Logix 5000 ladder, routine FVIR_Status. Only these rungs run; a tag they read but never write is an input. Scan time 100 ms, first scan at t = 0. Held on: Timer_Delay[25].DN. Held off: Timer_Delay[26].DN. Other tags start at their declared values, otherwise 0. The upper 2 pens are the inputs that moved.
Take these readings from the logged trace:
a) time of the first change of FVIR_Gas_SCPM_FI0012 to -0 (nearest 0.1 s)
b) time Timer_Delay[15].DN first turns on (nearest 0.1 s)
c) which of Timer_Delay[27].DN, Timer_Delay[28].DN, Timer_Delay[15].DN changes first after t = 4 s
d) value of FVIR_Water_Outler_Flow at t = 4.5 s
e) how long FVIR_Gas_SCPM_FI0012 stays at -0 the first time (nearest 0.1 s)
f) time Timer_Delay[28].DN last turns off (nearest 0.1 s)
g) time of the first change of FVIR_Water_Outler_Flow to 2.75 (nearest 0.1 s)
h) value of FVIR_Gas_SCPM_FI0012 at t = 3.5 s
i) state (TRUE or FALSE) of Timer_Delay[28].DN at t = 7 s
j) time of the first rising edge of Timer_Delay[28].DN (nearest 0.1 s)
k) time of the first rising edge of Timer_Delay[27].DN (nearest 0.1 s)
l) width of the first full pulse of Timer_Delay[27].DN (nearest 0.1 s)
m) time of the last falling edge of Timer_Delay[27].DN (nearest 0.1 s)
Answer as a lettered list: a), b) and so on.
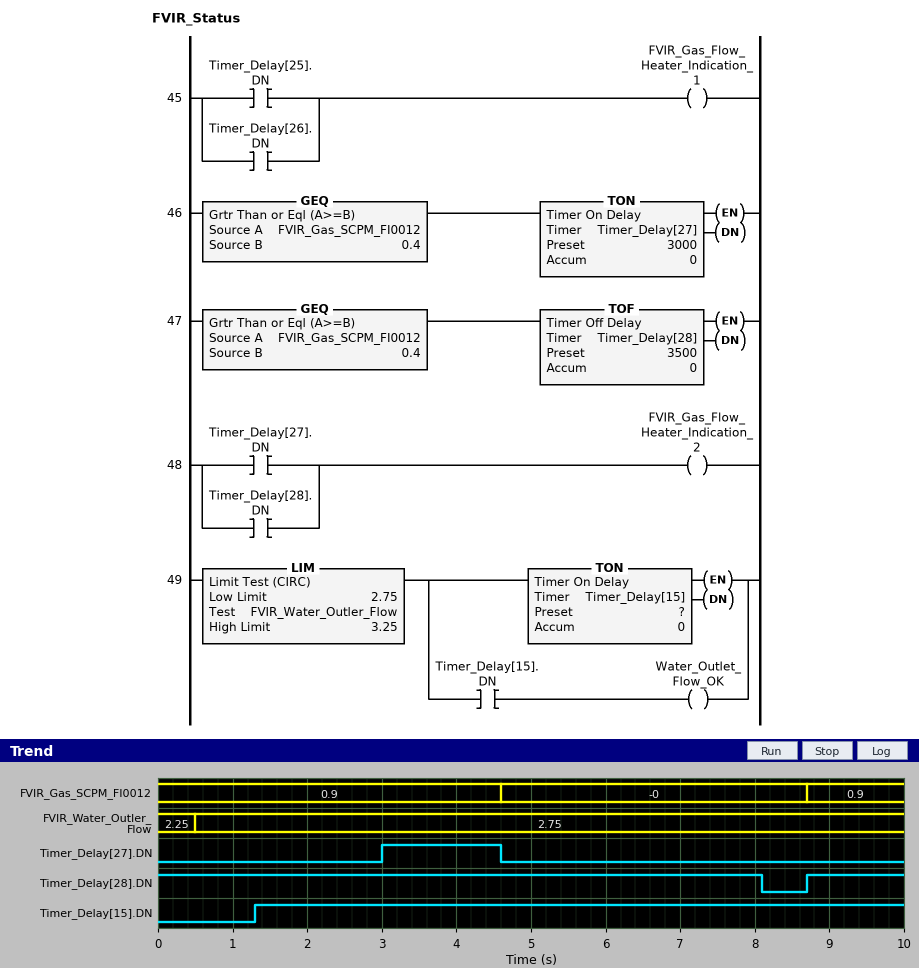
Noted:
a) 4.6 s
b) 1.3 s
c) Timer_Delay[27].DN
d) 2.75
e) 4.1 s
f) 8.1 s
g) 0.5 s
h) 0.9
i) TRUE
j) 8.7 s
k) 3.0 s
l) 1.6 s
m) 4.6 s
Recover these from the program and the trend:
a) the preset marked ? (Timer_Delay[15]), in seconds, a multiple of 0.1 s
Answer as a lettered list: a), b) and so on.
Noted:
a) 0.8 s
